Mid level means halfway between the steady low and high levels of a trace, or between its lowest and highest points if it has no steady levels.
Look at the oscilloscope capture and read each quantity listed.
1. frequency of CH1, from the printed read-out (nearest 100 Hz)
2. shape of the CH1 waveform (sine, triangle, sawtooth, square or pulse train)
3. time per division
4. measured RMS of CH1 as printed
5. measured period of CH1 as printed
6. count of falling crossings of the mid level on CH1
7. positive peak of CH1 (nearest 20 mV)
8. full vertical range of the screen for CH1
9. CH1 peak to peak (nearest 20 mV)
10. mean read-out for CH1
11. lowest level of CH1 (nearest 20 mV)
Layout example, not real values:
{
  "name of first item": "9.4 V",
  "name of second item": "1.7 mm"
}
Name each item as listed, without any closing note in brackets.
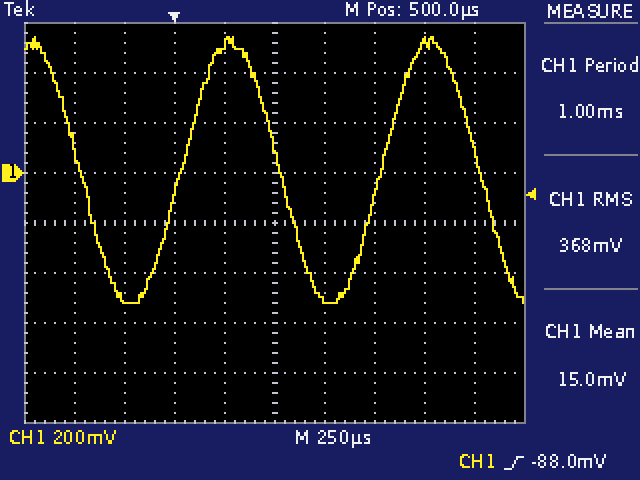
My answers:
{
  "frequency of CH1, from the printed read-out": "1.0 kHz",
  "shape of the CH1 waveform": "sine",
  "time per division": "250 µs",
  "measured RMS of CH1 as printed": "368 mV",
  "measured period of CH1 as printed": "1.00 ms",
  "count of falling crossings of the mid level on CH1": "3",
  "positive peak of CH1": "540 mV",
  "full vertical range of the screen for CH1": "1.6 V",
  "CH1 peak to peak": "1.06 V",
  "mean read-out for CH1": "15.0 mV",
  "lowest level of CH1": "-520 mV"
}
